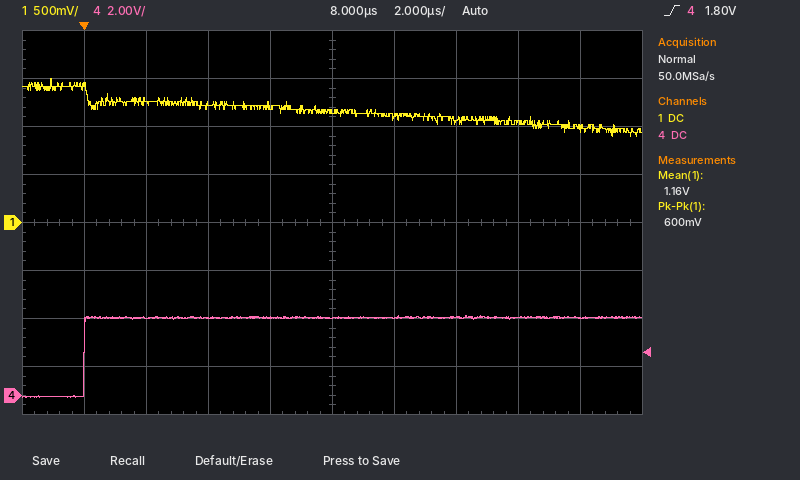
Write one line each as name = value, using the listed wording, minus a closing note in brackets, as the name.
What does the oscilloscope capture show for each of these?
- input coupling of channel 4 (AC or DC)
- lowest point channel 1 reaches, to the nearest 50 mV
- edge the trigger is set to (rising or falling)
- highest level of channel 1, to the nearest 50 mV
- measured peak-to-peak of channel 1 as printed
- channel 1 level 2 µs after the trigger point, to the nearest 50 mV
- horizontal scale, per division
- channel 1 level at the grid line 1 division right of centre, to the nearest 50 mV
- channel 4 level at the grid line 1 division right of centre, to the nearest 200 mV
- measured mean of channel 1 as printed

input coupling of channel 4 = DC
lowest point channel 1 reaches, to the nearest 50 mV = 900 mV
edge the trigger is set to = rising
highest level of channel 1, to the nearest 50 mV = 1.50 V
measured peak-to-peak of channel 1 as printed = 600 mV
channel 1 level 2 µs after the trigger point, to the nearest 50 mV = 1.25 V
horizontal scale, per division = 2 µs
channel 1 level at the grid line 1 division right of centre, to the nearest 50 mV = 1.10 V
channel 4 level at the grid line 1 division right of centre, to the nearest 200 mV = 3.2 V
measured mean of channel 1 as printed = 1.16 V
